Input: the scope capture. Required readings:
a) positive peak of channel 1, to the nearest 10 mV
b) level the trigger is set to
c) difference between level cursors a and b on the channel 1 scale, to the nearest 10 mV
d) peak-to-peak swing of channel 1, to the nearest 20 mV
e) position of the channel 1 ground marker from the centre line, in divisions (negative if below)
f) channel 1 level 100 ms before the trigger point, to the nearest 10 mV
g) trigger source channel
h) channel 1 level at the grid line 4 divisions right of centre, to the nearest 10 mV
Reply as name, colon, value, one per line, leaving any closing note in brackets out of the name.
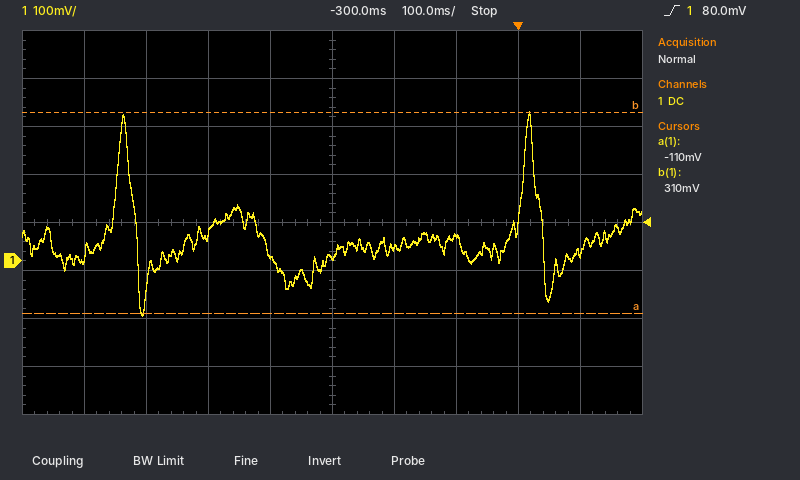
positive peak of channel 1, to the nearest 10 mV: 310 mV
level the trigger is set to: 80.0 mV
difference between level cursors a and b on the channel 1 scale, to the nearest 10 mV: 420 mV
peak-to-peak swing of channel 1, to the nearest 20 mV: 420 mV
position of the channel 1 ground marker from the centre line, in divisions: -0.8 div
channel 1 level 100 ms before the trigger point, to the nearest 10 mV: 50 mV
trigger source channel: channel 1
channel 1 level at the grid line 4 divisions right of centre, to the nearest 10 mV: 20 mV
